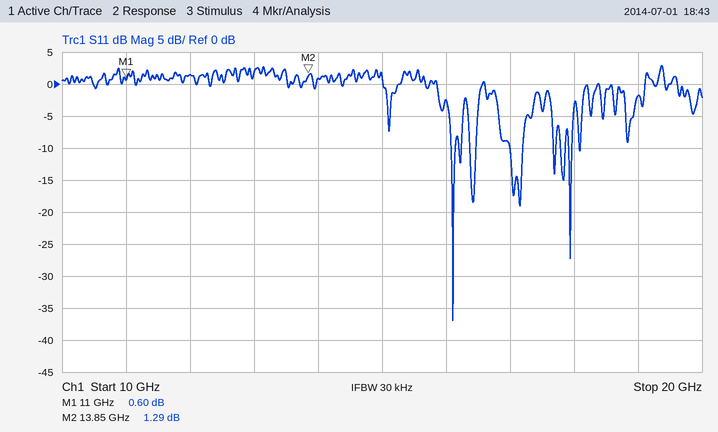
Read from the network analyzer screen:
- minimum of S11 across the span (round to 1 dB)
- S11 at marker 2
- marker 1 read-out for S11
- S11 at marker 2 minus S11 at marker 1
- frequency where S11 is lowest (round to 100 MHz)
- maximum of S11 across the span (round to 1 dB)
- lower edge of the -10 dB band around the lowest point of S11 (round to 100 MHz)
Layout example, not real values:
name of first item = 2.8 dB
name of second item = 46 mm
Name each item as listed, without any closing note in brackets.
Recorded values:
minimum of S11 across the span = -37 dB
S11 at marker 2 = 1.29 dB
marker 1 read-out for S11 = 0.60 dB
S11 at marker 2 minus S11 at marker 1 = 0.69 dB
frequency where S11 is lowest = 16.1 GHz
maximum of S11 across the span = 3 dB
lower edge of the -10 dB band around the lowest point of S11 = 16.1 GHz
